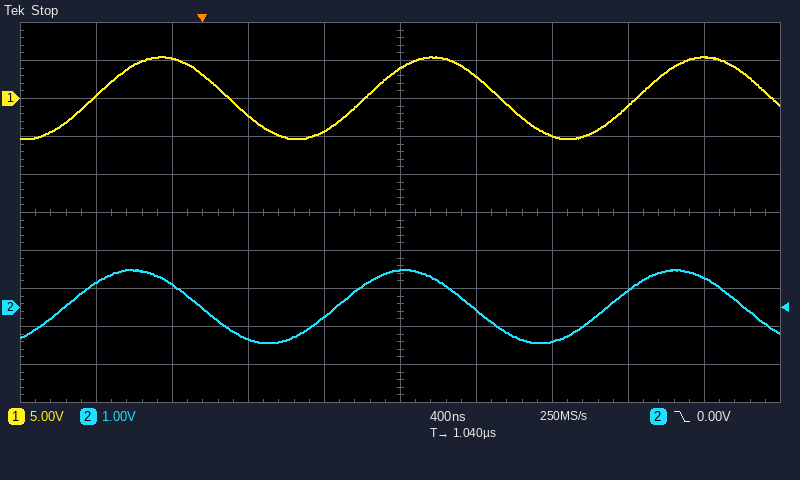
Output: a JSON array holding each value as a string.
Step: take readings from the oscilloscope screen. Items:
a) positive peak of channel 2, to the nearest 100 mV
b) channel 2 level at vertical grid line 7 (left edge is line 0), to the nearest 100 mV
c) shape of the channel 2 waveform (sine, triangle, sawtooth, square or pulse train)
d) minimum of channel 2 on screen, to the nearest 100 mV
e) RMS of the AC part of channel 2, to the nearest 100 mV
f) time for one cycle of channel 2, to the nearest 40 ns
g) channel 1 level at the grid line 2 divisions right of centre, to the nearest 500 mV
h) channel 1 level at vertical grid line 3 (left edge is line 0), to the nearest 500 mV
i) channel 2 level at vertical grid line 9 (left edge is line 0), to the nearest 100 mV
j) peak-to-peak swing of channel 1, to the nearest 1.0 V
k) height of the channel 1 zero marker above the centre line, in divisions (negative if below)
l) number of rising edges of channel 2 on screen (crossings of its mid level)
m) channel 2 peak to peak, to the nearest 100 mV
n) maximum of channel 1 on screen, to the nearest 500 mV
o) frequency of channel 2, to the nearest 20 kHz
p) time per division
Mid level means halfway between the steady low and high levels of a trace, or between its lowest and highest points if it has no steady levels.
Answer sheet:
["1.0 V", "-900 mV", "sine", "-900 mV", "700 mV", "1.44 µs", "-5.0 V", "-2.0 V", "800 mV", "11.0 V", "+3.0 div", "3", "1.9 V", "5.5 V", "700 kHz", "400 ns"]
